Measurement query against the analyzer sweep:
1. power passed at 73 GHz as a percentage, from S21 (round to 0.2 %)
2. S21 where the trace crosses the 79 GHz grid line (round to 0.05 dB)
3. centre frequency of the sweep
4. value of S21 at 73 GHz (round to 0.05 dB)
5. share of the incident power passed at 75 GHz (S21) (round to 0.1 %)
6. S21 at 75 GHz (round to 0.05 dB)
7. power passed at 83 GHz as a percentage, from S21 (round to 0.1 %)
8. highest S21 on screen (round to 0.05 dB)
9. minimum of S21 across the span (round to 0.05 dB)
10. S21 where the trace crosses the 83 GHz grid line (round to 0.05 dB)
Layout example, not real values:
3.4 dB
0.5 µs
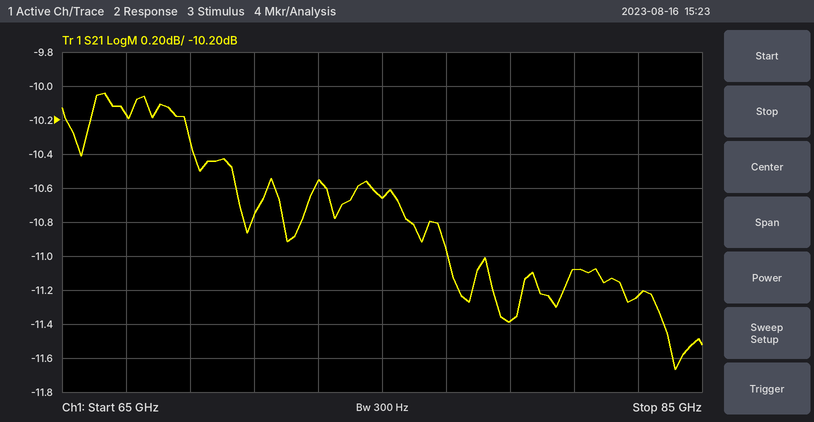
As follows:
8.8 %
-11.40 dB
75 GHz
-10.55 dB
8.6 %
-10.65 dB
7.5 %
-10.05 dB
-11.65 dB
-11.25 dB
